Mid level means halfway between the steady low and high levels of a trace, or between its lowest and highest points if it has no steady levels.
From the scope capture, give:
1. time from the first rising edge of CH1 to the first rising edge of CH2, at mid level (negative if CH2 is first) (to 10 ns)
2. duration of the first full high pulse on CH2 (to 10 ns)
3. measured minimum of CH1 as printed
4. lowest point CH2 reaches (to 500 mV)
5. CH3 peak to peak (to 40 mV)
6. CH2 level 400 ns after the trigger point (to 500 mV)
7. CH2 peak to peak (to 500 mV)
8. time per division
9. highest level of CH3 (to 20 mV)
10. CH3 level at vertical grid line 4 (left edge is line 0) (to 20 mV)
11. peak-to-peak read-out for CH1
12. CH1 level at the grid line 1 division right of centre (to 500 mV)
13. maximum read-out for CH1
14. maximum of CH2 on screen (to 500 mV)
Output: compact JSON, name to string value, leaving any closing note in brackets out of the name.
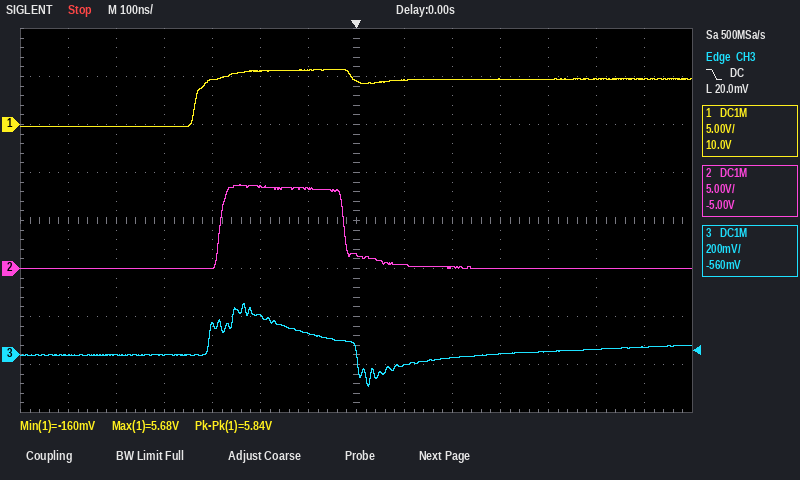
{"time from the first rising edge of CH1 to the first rising edge of CH2, at mid level (negative if CH2 is first)": "+50 ns", "duration of the first full high pulse on CH2": "260 ns", "measured minimum of CH1 as printed": "-160 mV", "lowest point CH2 reaches": "0.0 V", "CH3 peak to peak": "360 mV", "CH2 level 400 ns after the trigger point": "0.0 V", "CH2 peak to peak": "9.0 V", "time per division": "100 ns", "highest level of CH3": "220 mV", "CH3 level at vertical grid line 4 (left edge is line 0)": "120 mV", "peak-to-peak read-out for CH1": "5.84 V", "CH1 level at the grid line 1 division right of centre": "4.5 V", "maximum read-out for CH1": "5.68 V", "maximum of CH2 on screen": "9.0 V"}
